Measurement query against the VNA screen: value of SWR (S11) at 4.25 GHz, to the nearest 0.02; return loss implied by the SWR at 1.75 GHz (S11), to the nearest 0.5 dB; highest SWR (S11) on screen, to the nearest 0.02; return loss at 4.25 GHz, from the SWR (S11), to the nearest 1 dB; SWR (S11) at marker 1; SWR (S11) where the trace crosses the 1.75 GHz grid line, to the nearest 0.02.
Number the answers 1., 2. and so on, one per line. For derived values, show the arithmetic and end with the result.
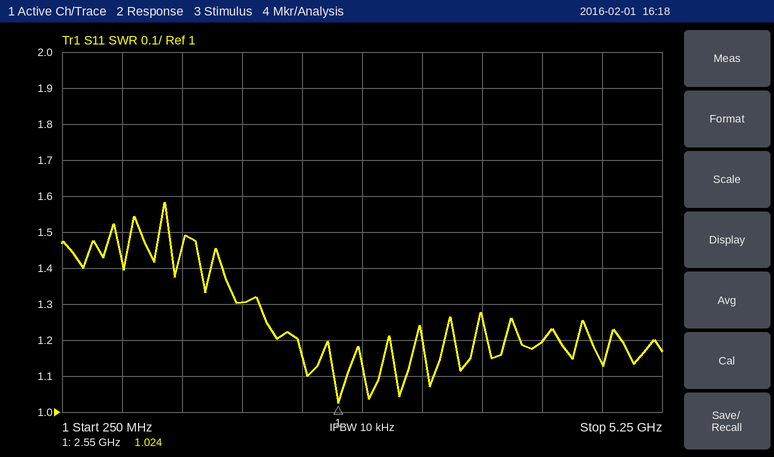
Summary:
1. 1.20
2. −20 log10((1.3 − 1)/(1.3 + 1)) ≈ 17.7 dB, so 17.5 dB to the nearest 0.5 dB
3. 1.58
4. −20 log10((1.2 − 1)/(1.2 + 1)) ≈ 21 dB
5. 1.024
6. 1.30
